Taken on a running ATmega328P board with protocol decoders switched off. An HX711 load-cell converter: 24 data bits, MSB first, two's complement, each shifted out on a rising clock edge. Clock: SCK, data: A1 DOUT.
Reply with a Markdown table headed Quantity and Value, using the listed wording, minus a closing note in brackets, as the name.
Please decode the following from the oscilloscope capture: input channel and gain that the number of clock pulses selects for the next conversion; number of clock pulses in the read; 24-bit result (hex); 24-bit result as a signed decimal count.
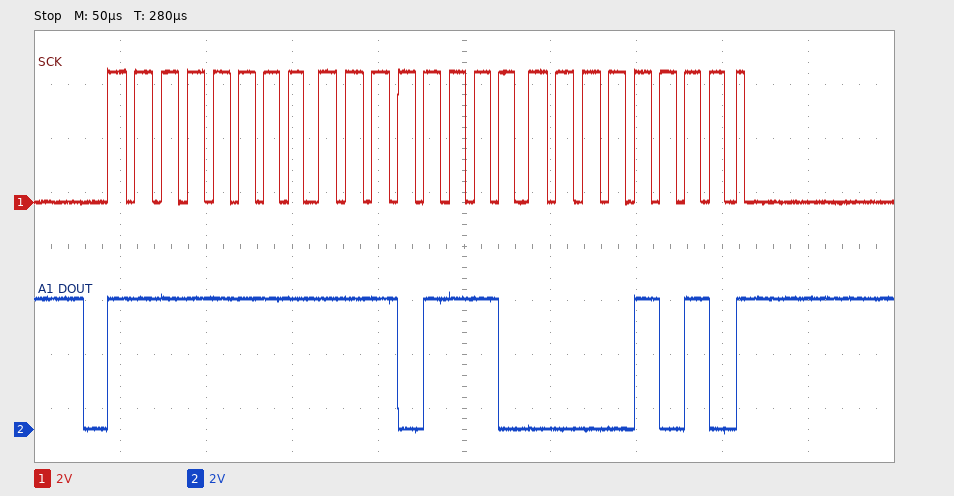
| Quantity | Value |
|---|---|
| input channel and gain that the number of clock pulses selects for the next conversion | channel A, gain 128 |
| number of clock pulses in the read | 25 |
| 24-bit result | 0xFFEE0A |
| 24-bit result as a signed decimal count | -4598 |
